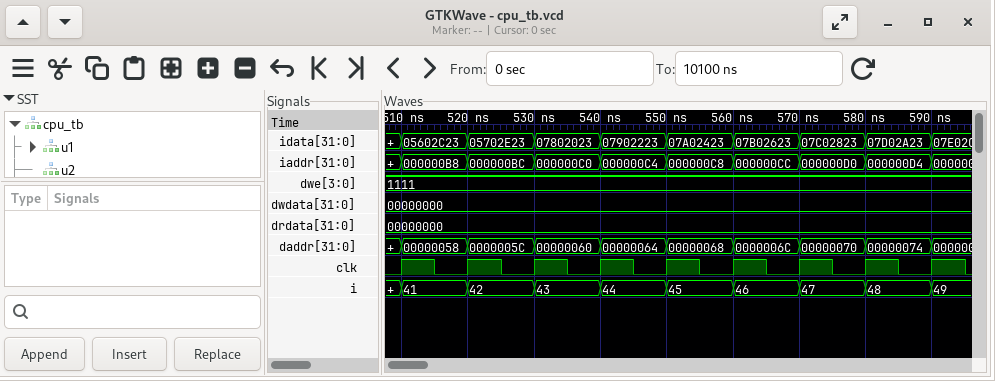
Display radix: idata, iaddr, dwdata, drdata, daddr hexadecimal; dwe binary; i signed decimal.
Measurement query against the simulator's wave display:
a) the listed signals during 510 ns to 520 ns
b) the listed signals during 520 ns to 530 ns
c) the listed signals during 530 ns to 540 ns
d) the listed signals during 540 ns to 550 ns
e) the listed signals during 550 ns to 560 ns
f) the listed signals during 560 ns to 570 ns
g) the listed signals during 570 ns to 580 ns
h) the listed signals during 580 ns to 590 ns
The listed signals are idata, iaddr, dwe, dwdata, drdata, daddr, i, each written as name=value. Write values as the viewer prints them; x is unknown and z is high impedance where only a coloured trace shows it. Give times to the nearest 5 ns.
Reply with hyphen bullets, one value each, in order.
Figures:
- idata=05602C23, iaddr=000000B8, dwe=1111, dwdata=00000000, drdata=00000000, daddr=00000058, i=41
- idata=05702E23, iaddr=000000BC, dwe=1111, dwdata=00000000, drdata=00000000, daddr=0000005C, i=42
- idata=07802023, iaddr=000000C0, dwe=1111, dwdata=00000000, drdata=00000000, daddr=00000060, i=43
- idata=07902223, iaddr=000000C4, dwe=1111, dwdata=00000000, drdata=00000000, daddr=00000064, i=44
- idata=07A02423, iaddr=000000C8, dwe=1111, dwdata=00000000, drdata=00000000, daddr=00000068, i=45
- idata=07B02623, iaddr=000000CC, dwe=1111, dwdata=00000000, drdata=00000000, daddr=0000006C, i=46
- idata=07C02823, iaddr=000000D0, dwe=1111, dwdata=00000000, drdata=00000000, daddr=00000070, i=47
- idata=07D02A23, iaddr=000000D4, dwe=1111, dwdata=00000000, drdata=00000000, daddr=00000074, i=48
